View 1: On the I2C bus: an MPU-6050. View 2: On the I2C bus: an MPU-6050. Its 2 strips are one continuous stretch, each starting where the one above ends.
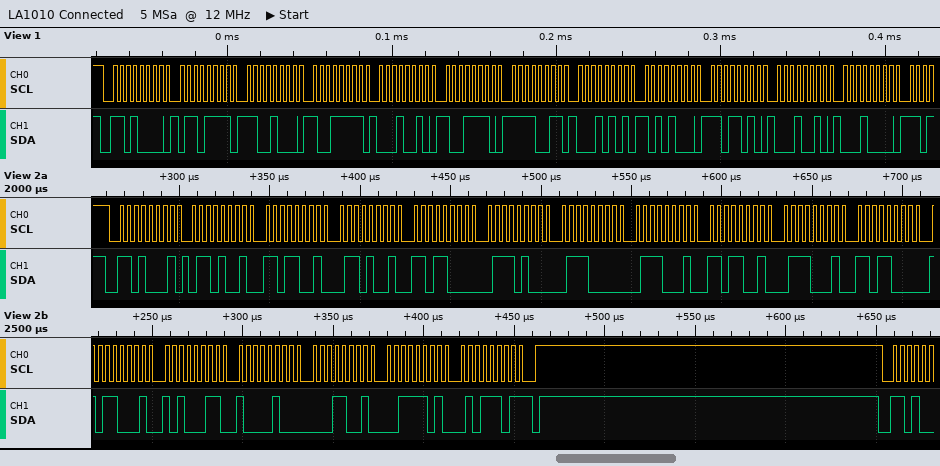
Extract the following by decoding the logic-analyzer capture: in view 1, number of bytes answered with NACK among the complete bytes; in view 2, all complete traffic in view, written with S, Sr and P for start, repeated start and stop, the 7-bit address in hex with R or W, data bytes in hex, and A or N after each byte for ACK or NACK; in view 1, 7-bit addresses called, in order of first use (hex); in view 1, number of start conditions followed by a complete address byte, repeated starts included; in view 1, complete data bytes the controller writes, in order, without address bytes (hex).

0
S 68R A 69 A D9 A 69 A D8 A 74 A 70 A 71 A D9 A 71 A D8 A B1 A A3 A 84 A 19 A 3D A 5D N P
0x68
1
6F C8 9F 12 9E F3 15 A8 DA 12 10
